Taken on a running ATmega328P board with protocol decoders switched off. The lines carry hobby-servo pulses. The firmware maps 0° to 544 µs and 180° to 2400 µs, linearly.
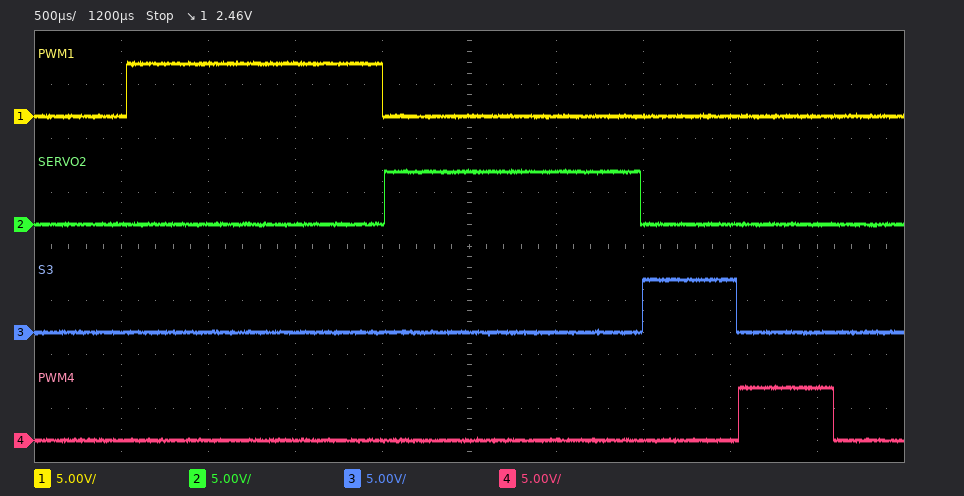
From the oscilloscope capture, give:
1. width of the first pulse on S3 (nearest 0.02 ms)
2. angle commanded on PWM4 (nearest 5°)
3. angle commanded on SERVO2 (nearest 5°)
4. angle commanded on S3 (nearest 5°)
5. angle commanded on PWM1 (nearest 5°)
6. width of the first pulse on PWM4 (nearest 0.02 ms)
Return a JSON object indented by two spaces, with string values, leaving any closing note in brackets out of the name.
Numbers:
{
  "width of the first pulse on S3": "0.54 ms",
  "angle commanded on PWM4": "0°",
  "angle commanded on SERVO2": "90°",
  "angle commanded on S3": "0°",
  "angle commanded on PWM1": "90°",
  "width of the first pulse on PWM4": "0.54 ms"
}
